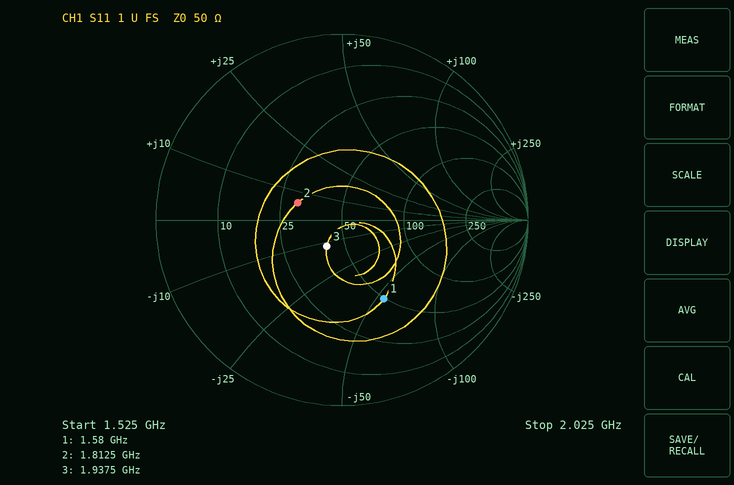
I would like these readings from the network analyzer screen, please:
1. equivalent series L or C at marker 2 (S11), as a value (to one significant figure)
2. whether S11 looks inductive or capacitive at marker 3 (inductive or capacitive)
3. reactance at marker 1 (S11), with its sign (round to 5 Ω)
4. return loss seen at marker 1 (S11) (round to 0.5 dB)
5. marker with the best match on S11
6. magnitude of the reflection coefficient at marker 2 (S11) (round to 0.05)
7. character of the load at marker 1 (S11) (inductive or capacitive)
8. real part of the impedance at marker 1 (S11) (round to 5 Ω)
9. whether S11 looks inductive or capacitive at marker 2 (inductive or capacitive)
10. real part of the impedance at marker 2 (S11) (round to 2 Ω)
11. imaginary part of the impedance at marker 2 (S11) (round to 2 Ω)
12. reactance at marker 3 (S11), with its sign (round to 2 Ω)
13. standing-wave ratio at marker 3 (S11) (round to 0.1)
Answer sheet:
500 pH
capacitive
-55 Ω
6.5 dB
marker 3
0.25
capacitive
50 Ω
inductive
30 Ω
+6 Ω
-12 Ω
1.4
